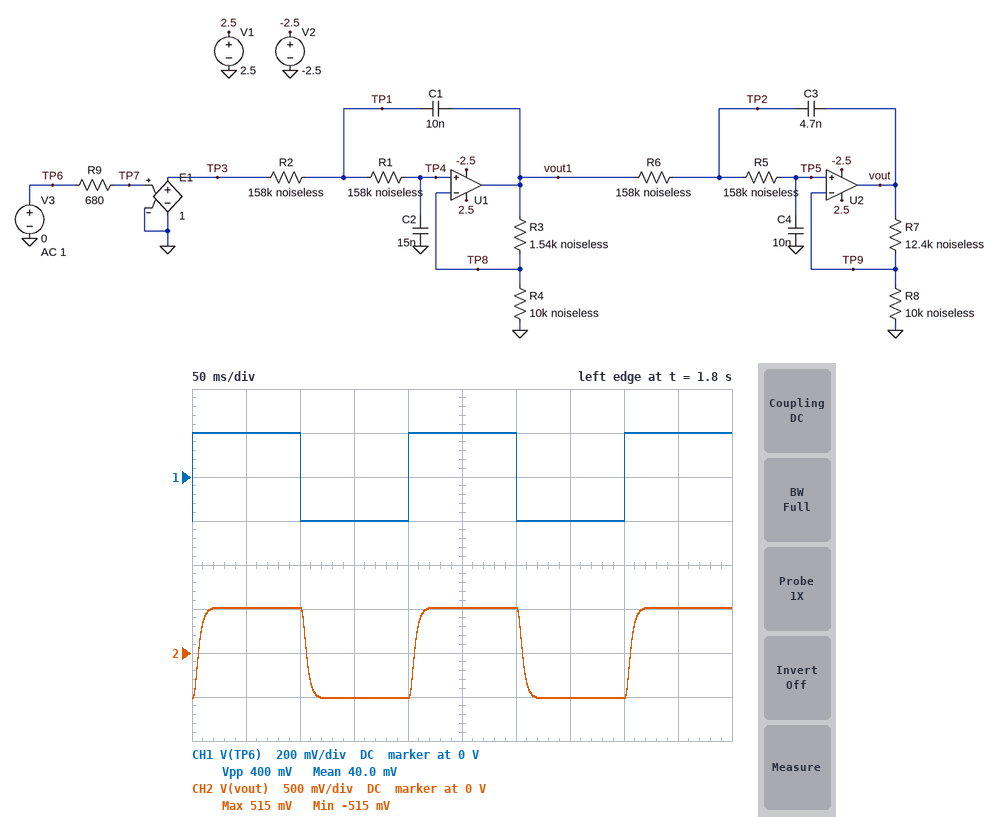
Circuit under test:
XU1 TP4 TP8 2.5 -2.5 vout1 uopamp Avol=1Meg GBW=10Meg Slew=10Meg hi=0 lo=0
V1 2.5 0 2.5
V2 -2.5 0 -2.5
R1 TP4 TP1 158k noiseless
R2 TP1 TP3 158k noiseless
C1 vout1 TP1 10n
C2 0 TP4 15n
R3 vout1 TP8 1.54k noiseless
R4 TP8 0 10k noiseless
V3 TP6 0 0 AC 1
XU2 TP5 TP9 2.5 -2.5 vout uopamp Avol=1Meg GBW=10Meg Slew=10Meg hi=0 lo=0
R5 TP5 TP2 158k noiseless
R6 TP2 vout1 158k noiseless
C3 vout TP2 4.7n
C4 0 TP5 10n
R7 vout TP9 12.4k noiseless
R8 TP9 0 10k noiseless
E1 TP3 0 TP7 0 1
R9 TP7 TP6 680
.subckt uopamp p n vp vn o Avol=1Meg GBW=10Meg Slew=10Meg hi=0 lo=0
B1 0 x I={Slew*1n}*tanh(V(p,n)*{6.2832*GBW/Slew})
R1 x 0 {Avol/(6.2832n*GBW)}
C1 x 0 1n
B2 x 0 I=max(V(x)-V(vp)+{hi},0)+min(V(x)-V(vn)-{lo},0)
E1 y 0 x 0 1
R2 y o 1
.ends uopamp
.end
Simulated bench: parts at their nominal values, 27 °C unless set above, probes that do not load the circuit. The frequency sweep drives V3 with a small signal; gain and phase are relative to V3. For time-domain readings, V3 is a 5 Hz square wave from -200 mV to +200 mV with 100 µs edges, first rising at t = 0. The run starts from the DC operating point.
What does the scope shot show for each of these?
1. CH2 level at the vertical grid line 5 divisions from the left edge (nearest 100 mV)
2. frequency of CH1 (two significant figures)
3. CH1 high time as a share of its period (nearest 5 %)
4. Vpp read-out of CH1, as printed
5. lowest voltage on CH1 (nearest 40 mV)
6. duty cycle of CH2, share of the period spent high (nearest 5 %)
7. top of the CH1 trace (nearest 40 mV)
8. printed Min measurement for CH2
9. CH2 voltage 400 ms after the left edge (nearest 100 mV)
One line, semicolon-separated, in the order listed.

500 mV; 5.0 Hz; 50 %; 400 mV; -200 mV; 50 %; 200 mV; -515 mV; -500 mV
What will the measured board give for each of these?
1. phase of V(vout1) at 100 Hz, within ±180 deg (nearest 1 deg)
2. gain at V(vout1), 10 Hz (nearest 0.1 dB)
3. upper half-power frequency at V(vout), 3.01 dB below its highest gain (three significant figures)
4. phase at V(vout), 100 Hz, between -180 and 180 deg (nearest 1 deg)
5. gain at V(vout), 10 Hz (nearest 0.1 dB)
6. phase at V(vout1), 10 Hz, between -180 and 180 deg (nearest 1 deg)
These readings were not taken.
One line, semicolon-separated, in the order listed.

-100 deg; 1.0 dB; 37.2 Hz; -169 deg; 8.0 dB; -16 deg
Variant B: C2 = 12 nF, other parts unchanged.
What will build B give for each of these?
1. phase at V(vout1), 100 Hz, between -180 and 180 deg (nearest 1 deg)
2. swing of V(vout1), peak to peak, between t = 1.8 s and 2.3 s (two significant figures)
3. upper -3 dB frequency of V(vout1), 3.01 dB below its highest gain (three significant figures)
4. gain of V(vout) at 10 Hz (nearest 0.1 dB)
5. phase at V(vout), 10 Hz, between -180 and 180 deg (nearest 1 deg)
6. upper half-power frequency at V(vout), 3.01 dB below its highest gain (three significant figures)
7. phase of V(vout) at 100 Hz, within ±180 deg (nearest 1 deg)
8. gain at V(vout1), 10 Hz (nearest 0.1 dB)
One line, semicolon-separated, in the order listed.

-95 deg; 460 mV; 57.1 Hz; 8.1 dB; -21 deg; 46.2 Hz; -164 deg; 1.1 dB
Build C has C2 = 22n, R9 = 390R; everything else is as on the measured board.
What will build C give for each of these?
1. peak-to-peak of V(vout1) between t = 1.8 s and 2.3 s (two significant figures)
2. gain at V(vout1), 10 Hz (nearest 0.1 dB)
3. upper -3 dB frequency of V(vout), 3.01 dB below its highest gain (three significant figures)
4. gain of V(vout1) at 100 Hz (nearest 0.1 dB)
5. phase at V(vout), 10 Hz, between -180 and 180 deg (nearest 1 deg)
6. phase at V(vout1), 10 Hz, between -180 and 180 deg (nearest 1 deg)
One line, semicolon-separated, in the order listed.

460 mV; 0.7 dB; 25.2 Hz; -11.6 dB; -31 deg; -23 deg
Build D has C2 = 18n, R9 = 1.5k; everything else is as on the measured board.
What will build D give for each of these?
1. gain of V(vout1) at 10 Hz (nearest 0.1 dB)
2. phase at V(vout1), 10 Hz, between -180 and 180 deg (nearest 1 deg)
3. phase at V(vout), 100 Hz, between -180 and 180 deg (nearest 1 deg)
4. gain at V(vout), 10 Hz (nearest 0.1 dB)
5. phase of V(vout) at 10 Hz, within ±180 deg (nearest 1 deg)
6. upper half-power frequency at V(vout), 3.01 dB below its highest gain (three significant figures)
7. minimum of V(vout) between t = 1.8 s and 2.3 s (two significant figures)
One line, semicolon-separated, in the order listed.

0.9 dB; -19 deg; -172 deg; 7.9 dB; -27 deg; 31.0 Hz; -520 mV
